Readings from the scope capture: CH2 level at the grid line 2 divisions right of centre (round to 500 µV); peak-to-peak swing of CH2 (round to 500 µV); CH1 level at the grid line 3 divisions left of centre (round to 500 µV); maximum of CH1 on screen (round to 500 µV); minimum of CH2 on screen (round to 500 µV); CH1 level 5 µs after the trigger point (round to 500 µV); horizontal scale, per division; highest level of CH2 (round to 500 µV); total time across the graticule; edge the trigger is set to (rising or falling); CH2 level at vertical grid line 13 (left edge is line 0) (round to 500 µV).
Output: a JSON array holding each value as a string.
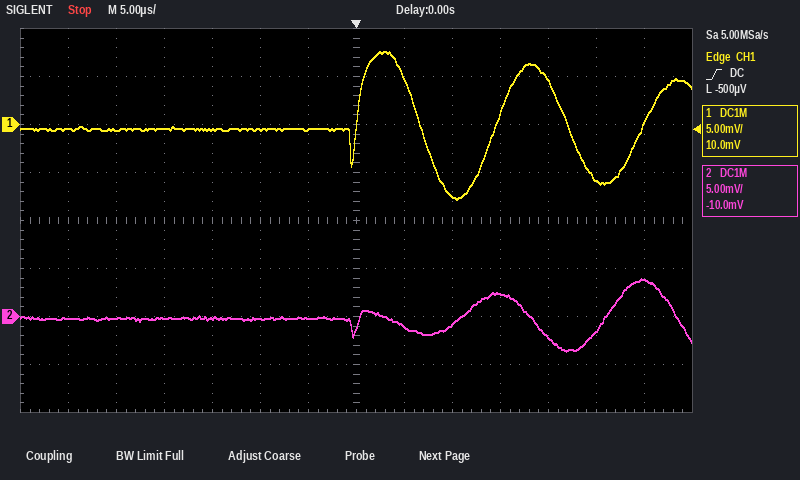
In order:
["-1.0 mV", "7.5 mV", "-500 µV", "7.5 mV", "-3.5 mV", "5.0 mV", "5 µs", "4.0 mV", "70 µs", "rising", "4.0 mV"]
